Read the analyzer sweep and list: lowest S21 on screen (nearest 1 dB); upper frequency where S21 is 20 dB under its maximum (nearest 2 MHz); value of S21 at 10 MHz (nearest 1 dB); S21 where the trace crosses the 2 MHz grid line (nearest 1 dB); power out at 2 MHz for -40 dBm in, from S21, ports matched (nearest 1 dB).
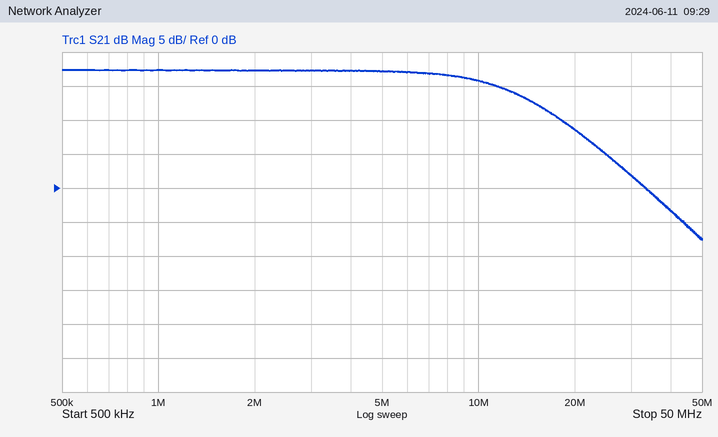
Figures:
-8 dB
38 MHz
16 dB
17 dB
-23 dBm
